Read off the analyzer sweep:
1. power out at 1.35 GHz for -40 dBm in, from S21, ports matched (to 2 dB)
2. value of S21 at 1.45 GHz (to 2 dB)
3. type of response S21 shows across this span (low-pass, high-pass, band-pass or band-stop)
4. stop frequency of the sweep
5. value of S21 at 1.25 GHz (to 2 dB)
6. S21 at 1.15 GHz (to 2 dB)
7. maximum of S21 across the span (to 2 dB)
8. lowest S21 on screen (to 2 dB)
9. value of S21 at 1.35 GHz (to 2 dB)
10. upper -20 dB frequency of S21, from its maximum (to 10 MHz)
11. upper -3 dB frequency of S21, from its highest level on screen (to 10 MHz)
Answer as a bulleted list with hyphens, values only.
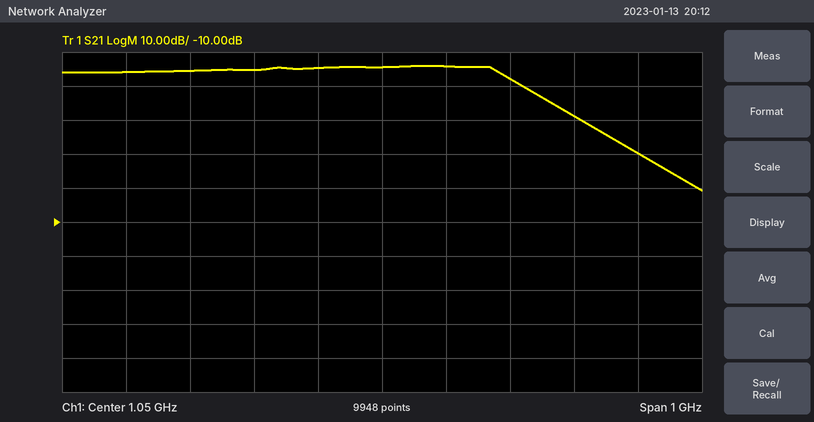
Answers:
- -18 dBm
- 10 dB
- low-pass
- 1.55 GHz
- 32 dB
- 36 dB
- 36 dB
- 0 dB
- 22 dB
- 1.40 GHz
- 1.24 GHz
